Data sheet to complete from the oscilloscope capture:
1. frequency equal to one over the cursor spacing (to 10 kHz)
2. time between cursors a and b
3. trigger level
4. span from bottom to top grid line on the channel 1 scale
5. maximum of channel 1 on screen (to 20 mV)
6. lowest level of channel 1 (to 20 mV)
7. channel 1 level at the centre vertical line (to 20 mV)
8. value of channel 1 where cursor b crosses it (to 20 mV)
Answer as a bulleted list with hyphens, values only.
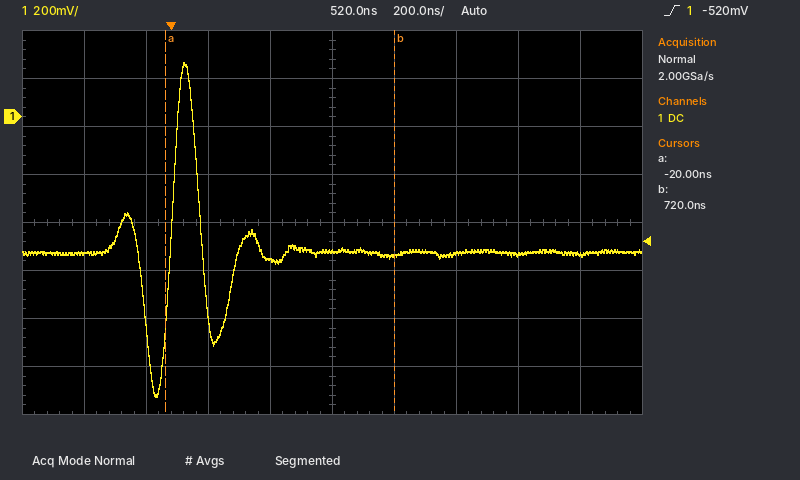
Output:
- 1.35 MHz
- 740 ns
- -520 mV
- 1.6 V
- 220 mV
- -1.16 V
- -560 mV
- -580 mV
